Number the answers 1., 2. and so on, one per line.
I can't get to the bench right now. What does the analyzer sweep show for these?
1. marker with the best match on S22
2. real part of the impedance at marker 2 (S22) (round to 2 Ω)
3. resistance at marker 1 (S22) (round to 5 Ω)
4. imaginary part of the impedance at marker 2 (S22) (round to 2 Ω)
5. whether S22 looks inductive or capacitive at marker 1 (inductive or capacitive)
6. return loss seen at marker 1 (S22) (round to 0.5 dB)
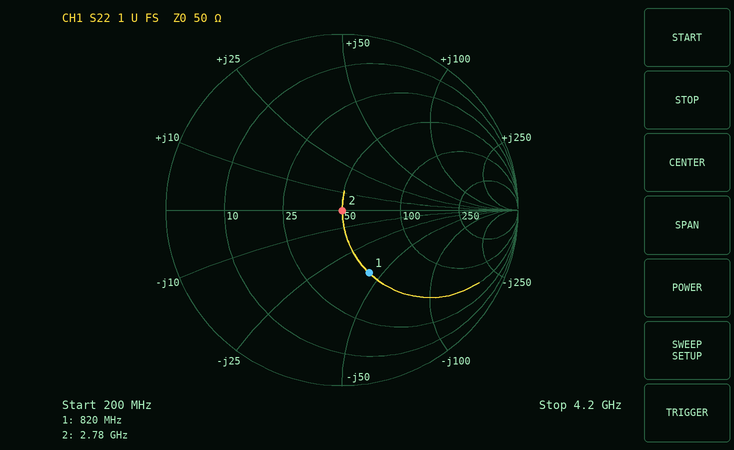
1. marker 2
2. 50 Ω
3. 50 Ω
4. 0 Ω
5. capacitive
6. 8.0 dB
